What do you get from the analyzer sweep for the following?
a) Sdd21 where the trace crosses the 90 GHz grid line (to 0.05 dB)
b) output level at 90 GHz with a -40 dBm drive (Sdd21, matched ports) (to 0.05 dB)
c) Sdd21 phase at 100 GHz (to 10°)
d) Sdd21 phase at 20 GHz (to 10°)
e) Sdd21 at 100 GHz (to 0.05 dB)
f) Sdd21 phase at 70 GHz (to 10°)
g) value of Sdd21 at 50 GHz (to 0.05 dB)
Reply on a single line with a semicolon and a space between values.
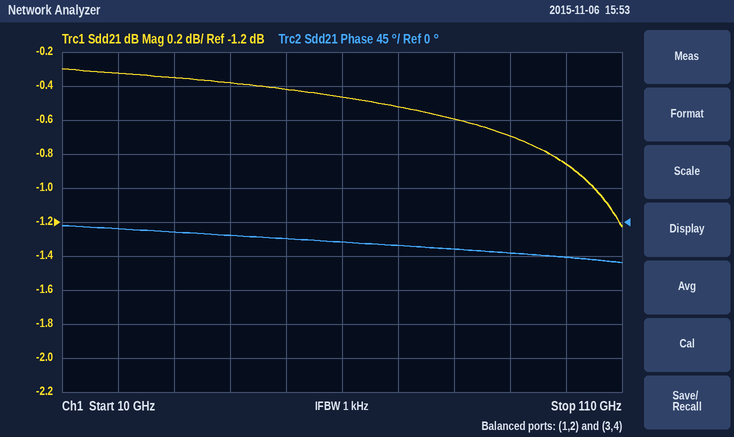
-0.70 dB; -40.70 dBm; -50°; -10°; -0.85 dB; -30°; -0.40 dB
